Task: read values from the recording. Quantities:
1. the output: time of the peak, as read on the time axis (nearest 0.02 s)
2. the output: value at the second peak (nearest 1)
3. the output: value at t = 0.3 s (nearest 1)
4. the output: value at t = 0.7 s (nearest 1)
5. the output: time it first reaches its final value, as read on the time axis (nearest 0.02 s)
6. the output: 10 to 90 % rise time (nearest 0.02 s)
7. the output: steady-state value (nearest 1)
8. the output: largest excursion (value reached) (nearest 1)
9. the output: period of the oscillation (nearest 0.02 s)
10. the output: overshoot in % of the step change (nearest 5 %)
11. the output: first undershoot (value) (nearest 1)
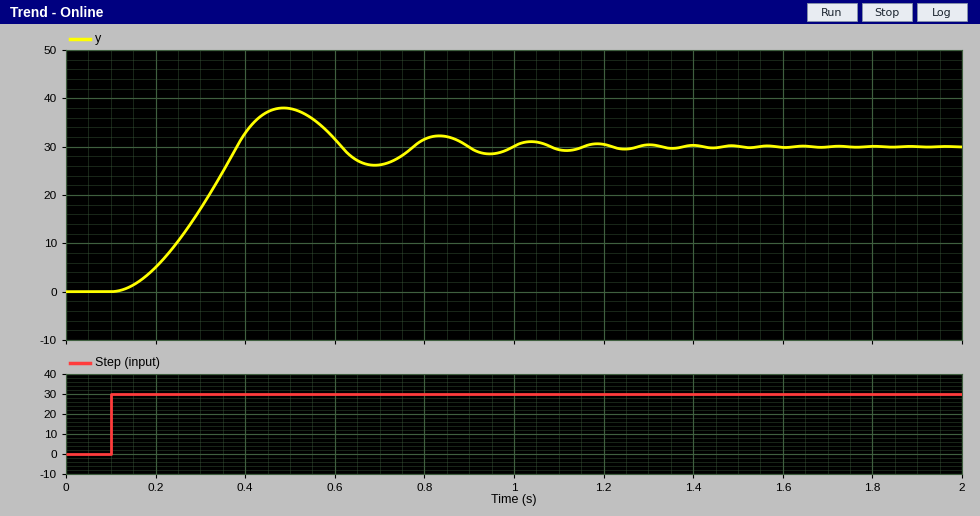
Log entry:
0.48 s
32
17
26
0.38 s
0.18 s
30
38
0.34 s
25 %
26
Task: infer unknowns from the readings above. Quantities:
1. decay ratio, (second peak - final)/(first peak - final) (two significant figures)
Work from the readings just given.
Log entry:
0.25
